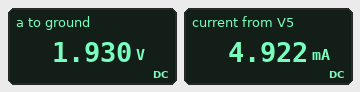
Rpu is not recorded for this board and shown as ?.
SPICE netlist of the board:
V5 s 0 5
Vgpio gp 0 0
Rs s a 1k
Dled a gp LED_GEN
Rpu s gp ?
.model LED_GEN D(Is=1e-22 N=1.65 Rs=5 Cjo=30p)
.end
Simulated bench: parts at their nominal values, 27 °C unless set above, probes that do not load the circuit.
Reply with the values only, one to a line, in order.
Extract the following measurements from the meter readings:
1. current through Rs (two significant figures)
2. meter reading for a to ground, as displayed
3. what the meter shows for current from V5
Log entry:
3.1 mA
1.930 V
4.922 mA
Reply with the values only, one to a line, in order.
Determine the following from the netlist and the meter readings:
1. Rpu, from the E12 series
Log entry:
2.7 kΩ
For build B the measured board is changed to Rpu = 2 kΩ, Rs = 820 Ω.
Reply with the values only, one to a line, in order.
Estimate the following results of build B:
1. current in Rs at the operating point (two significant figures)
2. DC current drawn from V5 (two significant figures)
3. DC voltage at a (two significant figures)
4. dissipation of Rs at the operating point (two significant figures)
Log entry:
3.7 mA
6.2 mA
1.9 V
11 mW
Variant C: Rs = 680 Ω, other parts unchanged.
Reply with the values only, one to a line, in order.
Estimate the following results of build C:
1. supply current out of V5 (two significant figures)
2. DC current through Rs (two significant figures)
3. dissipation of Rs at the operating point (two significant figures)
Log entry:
6.3 mA
4.5 mA
14 mW
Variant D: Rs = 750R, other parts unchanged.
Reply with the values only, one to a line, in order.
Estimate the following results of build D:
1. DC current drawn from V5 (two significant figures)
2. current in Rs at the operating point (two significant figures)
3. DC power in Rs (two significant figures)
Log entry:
5.9 mA
4.1 mA
12 mW
